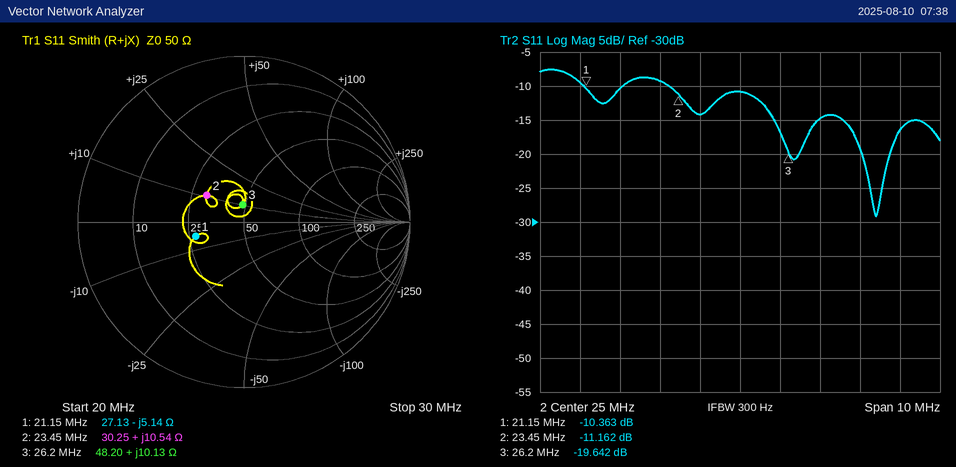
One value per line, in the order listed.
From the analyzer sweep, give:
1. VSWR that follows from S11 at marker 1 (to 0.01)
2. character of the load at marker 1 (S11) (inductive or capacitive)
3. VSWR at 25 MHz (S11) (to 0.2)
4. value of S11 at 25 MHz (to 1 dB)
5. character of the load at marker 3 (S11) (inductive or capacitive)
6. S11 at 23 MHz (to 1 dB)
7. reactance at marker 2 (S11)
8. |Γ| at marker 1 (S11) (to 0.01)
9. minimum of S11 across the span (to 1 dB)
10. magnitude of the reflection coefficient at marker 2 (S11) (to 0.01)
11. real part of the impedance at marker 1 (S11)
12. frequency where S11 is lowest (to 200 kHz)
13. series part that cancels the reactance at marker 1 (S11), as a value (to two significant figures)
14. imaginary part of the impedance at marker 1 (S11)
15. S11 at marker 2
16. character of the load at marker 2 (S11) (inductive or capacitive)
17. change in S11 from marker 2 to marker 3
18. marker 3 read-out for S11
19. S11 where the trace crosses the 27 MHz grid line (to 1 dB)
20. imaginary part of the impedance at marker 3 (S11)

1.87
capacitive
1.8
-11 dB
inductive
-9 dB
+10.54 Ω
0.30
-29 dB
0.28
27.13 Ω
28.4 MHz
39 nH
-5.14 Ω
-11.162 dB
inductive
-8.480 dB
-19.642 dB
-15 dB
+10.13 Ω
